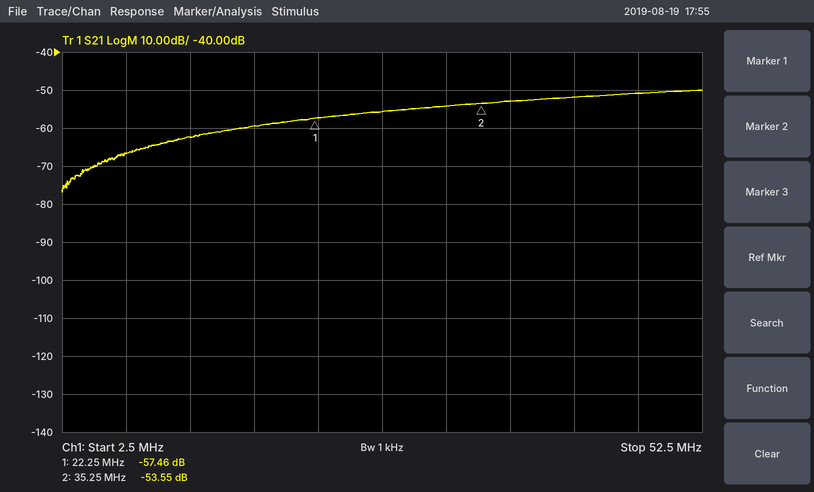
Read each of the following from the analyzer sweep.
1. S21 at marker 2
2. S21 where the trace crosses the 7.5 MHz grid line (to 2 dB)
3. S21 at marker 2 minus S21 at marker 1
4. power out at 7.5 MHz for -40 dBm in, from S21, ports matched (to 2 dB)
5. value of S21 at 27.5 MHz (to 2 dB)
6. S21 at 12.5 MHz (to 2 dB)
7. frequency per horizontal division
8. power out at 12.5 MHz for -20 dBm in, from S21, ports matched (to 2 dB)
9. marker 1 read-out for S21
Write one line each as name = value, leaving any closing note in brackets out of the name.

S21 at marker 2 = -53.55 dB
S21 where the trace crosses the 7.5 MHz grid line = -66 dB
S21 at marker 2 minus S21 at marker 1 = 3.91 dB
power out at 7.5 MHz for -40 dBm in, from S21, ports matched = -106 dBm
value of S21 at 27.5 MHz = -56 dB
S21 at 12.5 MHz = -62 dB
frequency per horizontal division = 5 MHz
power out at 12.5 MHz for -20 dBm in, from S21, ports matched = -82 dBm
marker 1 read-out for S21 = -57.46 dB
